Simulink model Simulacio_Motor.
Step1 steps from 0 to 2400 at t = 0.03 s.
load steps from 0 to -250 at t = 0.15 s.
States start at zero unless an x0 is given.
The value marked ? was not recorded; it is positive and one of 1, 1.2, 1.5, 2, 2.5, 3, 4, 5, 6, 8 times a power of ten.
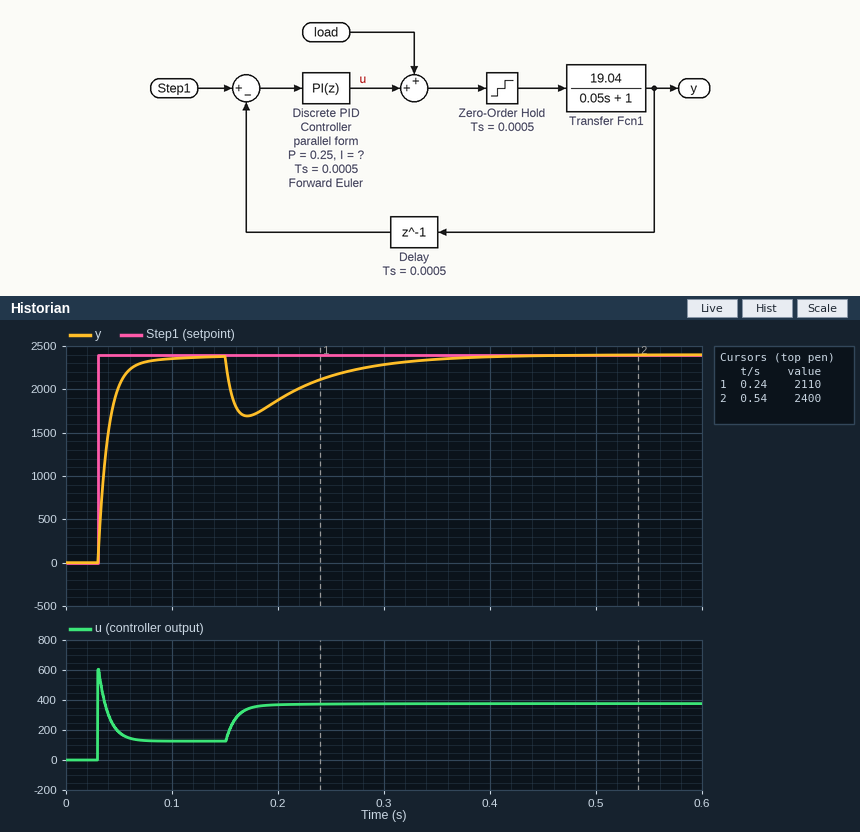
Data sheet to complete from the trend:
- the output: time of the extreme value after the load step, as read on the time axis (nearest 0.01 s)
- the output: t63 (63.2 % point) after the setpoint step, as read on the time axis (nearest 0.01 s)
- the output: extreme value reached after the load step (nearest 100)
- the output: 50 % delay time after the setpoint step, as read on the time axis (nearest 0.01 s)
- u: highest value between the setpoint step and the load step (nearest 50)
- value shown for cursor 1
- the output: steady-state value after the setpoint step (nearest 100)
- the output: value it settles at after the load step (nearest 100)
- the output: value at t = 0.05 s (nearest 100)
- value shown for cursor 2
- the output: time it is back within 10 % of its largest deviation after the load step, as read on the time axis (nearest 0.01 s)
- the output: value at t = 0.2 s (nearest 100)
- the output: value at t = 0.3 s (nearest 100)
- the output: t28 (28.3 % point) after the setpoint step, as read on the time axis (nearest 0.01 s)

0.17 s
0.04 s
1700
0.04 s
600
2110
2400
2400
2000
2400
0.33 s
1900
2300
0.03 s
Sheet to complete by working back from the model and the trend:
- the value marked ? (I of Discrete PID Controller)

4
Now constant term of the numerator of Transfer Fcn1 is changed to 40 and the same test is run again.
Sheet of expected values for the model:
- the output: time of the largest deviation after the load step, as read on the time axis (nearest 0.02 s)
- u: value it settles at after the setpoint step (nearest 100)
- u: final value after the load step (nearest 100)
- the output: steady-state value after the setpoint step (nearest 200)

0.16 s
100
300
2400
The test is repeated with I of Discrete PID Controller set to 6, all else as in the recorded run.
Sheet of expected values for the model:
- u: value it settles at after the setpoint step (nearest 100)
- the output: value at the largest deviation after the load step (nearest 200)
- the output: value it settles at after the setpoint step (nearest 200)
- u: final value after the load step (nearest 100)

100
1800
2400
400
